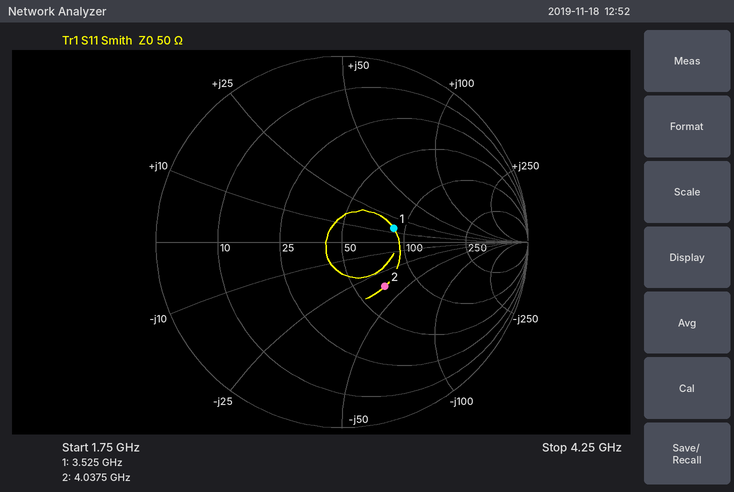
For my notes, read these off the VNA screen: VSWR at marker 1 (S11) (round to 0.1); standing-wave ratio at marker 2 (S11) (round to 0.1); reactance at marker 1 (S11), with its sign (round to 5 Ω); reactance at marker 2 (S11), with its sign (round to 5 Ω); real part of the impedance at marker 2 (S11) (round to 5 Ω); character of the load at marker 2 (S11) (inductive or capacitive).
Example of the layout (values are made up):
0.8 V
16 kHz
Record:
1.8
2.0
+15 Ω
-35 Ω
70 Ω
capacitive
